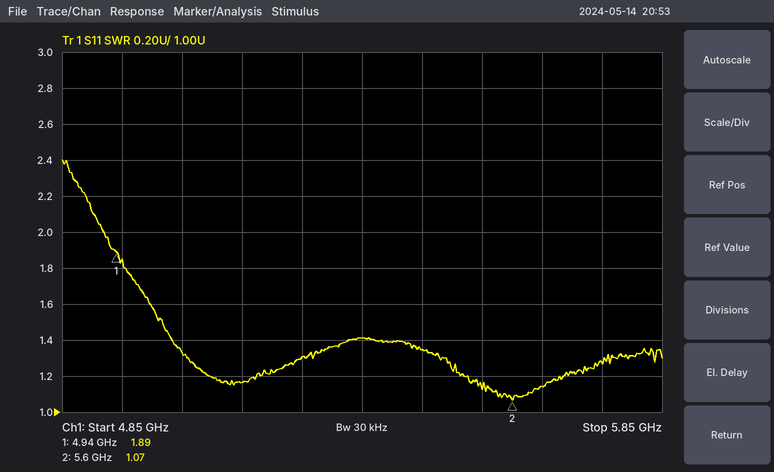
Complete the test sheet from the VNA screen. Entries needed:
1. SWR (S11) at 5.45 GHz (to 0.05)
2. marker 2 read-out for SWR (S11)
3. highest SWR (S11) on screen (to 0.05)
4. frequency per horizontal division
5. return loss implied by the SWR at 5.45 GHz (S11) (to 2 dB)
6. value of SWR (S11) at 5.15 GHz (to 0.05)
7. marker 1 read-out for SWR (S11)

1.35
1.07
2.40
100 MHz
16 dB
1.15
1.89
